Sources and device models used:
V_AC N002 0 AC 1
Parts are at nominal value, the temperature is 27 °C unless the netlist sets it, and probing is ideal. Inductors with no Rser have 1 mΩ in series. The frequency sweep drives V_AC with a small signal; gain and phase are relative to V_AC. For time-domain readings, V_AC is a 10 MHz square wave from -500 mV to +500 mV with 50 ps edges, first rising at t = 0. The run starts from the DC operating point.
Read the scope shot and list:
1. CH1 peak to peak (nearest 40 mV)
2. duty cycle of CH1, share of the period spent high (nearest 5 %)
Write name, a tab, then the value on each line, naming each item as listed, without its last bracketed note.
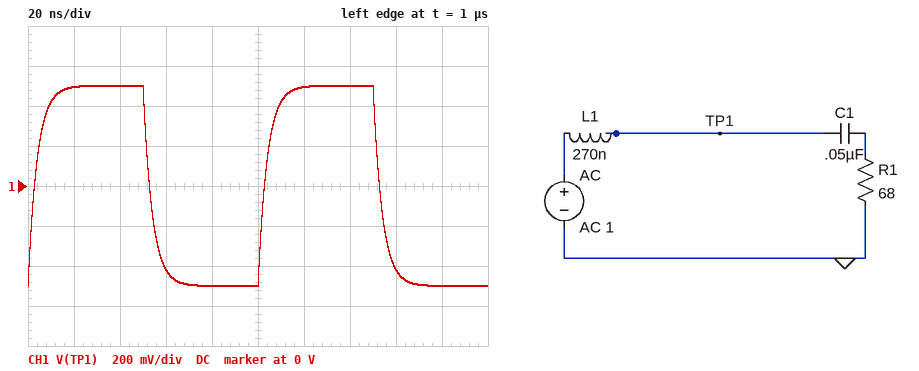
CH1 peak to peak	1.00 V
duty cycle of CH1, share of the period spent high	50 %
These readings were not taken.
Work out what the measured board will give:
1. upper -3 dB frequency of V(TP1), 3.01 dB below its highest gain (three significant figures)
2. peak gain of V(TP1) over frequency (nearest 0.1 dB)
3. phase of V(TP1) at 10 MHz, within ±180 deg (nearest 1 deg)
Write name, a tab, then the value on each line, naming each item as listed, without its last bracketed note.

upper -3 dB frequency of V(TP1), 3.01 dB below its highest gain	40.0 MHz
peak gain of V(TP1) over frequency	0 dB
phase of V(TP1) at 10 MHz, within ±180 deg	-14 deg
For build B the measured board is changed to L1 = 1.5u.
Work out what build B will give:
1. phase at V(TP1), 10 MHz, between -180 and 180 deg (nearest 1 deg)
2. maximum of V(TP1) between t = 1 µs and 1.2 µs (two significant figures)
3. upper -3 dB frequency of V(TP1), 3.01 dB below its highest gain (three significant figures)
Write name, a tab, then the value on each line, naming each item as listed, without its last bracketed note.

phase at V(TP1), 10 MHz, between -180 and 180 deg	-54 deg
maximum of V(TP1) between t = 1 µs and 1.2 µs	410 mV
upper -3 dB frequency of V(TP1), 3.01 dB below its highest gain	7.18 MHz
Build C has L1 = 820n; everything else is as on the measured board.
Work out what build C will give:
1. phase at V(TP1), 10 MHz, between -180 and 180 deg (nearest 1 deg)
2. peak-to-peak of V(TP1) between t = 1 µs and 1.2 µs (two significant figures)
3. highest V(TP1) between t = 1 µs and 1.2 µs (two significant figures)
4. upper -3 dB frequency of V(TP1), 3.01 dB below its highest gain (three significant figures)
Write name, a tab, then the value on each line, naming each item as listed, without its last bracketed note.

phase at V(TP1), 10 MHz, between -180 and 180 deg	-37 deg
peak-to-peak of V(TP1) between t = 1 µs and 1.2 µs	970 mV
highest V(TP1) between t = 1 µs and 1.2 µs	490 mV
upper -3 dB frequency of V(TP1), 3.01 dB below its highest gain	13.2 MHz
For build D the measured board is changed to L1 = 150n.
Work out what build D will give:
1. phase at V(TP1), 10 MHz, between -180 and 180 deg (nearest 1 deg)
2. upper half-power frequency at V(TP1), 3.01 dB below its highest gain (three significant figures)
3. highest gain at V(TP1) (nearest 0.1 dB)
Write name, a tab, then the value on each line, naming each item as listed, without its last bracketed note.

phase at V(TP1), 10 MHz, between -180 and 180 deg	-8 deg
upper half-power frequency at V(TP1), 3.01 dB below its highest gain	72.1 MHz
highest gain at V(TP1)	0 dB
